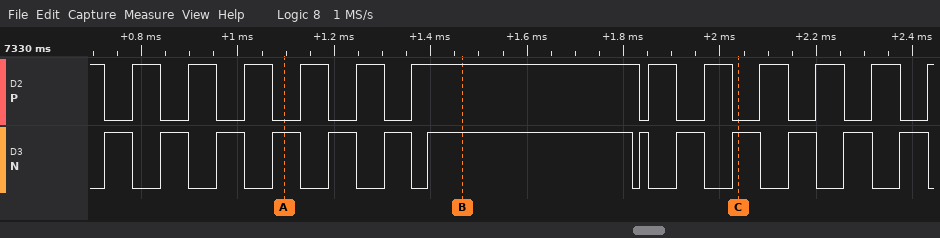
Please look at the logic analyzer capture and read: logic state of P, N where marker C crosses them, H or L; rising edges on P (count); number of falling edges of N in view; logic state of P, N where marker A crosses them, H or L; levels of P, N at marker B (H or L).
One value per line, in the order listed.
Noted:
P=L, N=H
12
13
P=L, N=H
P=H, N=H
